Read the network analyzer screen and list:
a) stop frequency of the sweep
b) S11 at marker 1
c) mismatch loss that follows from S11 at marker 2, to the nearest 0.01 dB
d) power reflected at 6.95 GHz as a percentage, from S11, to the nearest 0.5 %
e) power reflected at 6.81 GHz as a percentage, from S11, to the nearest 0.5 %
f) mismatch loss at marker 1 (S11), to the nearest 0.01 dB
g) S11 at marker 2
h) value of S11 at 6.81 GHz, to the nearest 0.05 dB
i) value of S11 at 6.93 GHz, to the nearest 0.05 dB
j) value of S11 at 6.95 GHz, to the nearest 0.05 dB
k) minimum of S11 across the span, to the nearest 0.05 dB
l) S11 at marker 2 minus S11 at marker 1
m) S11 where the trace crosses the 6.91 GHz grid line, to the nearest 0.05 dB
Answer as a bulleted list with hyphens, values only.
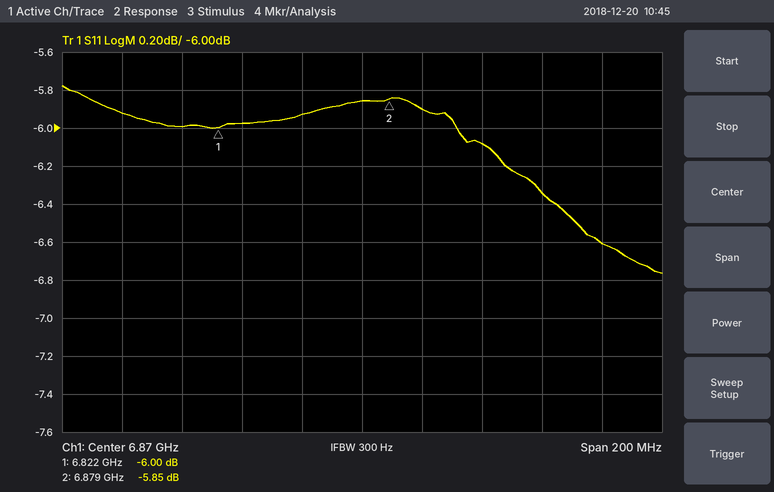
- 6.97 GHz
- -6.00 dB
- 1.31 dB
- 22.0 %
- 25.0 %
- 1.26 dB
- -5.85 dB
- -6.00 dB
- -6.35 dB
- -6.60 dB
- -6.75 dB
- 0.15 dB
- -6.10 dB
